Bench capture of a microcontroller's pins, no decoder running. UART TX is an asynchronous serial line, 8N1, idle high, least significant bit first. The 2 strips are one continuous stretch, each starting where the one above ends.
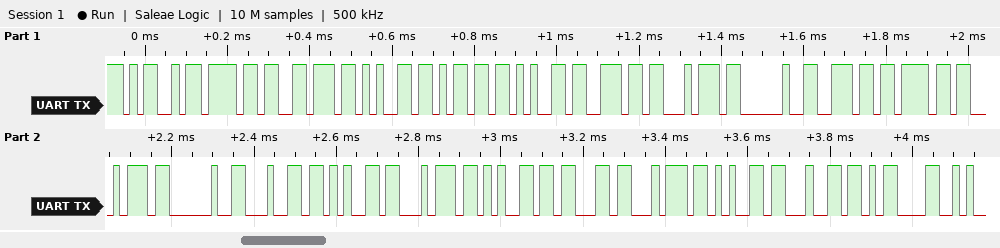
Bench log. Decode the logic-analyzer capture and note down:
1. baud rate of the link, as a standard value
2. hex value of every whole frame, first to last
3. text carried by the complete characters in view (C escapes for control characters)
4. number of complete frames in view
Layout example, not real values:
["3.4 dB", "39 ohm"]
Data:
["57600 baud", "4D 6F 76 65 6D 65 6E 74 20 6E 6F 74 20 64 65 74 65 63 74 65 64 0D", "\"Movement not detected\\r\"", "22"]
